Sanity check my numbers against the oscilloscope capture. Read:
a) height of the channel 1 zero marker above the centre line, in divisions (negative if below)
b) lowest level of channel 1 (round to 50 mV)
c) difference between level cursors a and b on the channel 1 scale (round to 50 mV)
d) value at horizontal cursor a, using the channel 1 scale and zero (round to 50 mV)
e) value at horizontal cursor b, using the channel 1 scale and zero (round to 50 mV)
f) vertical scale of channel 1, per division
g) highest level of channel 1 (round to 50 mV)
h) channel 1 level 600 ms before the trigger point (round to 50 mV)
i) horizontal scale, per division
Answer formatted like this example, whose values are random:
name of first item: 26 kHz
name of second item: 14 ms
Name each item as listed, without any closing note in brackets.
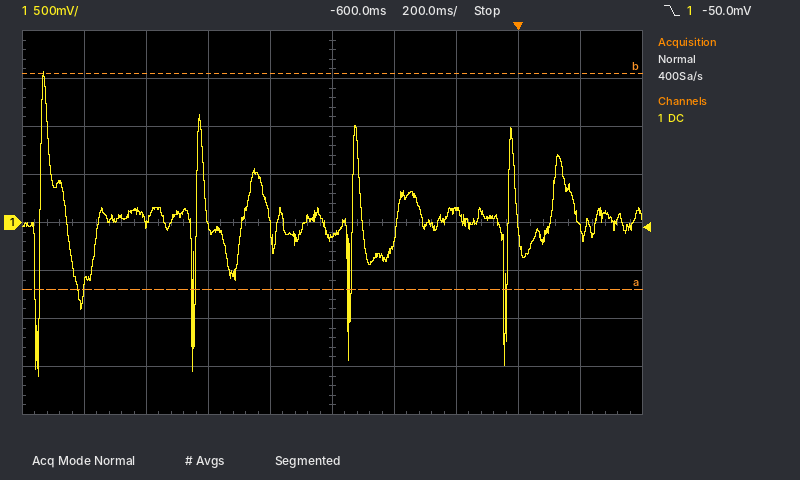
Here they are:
height of the channel 1 zero marker above the centre line, in divisions: 0.0 div
lowest level of channel 1: -1.60 V
difference between level cursors a and b on the channel 1 scale: 2.25 V
value at horizontal cursor a, using the channel 1 scale and zero: -700 mV
value at horizontal cursor b, using the channel 1 scale and zero: 1.55 V
vertical scale of channel 1, per division: 500 mV
highest level of channel 1: 1.55 V
channel 1 level 600 ms before the trigger point: -150 mV
horizontal scale, per division: 200 ms
